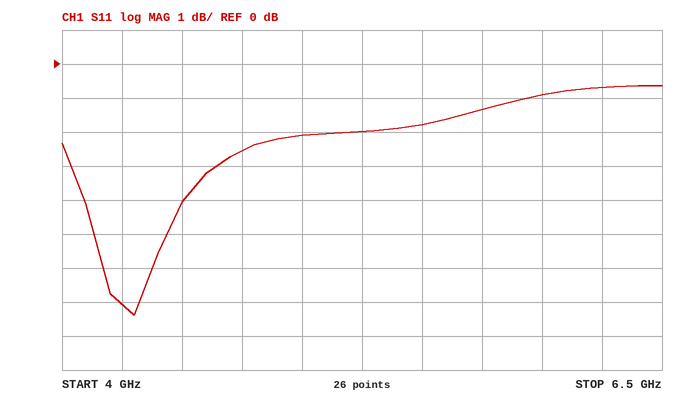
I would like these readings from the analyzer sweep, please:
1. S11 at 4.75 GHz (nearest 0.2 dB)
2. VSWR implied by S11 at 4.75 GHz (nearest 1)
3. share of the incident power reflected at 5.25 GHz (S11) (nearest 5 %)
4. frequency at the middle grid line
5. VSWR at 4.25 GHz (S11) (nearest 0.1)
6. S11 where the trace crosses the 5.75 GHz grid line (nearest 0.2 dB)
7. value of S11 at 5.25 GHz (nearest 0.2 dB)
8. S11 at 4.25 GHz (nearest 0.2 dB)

-2.6 dB
7
65 %
5.25 GHz
2.6
-1.4 dB
-2.0 dB
-7.0 dB
